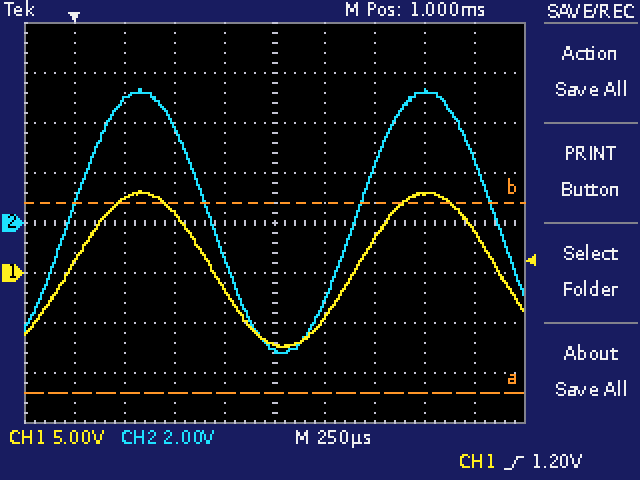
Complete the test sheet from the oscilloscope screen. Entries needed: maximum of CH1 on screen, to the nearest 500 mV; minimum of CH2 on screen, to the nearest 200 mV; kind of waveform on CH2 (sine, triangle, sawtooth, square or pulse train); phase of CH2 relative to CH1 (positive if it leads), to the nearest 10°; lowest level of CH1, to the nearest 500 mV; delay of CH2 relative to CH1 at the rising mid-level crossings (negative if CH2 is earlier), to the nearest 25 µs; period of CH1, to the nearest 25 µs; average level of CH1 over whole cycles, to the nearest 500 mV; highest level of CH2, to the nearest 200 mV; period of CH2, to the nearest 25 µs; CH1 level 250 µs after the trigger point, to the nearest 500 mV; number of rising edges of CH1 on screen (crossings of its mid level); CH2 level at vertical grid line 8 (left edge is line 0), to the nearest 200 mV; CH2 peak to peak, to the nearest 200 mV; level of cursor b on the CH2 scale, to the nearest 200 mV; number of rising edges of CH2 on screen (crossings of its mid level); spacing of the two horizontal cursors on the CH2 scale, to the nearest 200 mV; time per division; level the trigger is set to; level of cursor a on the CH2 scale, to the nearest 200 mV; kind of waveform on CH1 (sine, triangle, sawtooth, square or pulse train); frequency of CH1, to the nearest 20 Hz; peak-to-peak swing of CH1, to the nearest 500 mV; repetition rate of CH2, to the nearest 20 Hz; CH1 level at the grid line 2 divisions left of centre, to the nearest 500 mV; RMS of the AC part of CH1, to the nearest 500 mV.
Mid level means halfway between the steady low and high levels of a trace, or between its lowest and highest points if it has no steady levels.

8.0 V
-5.2 V
sine
0°
-7.5 V
0 µs
1.425 ms
500 mV
5.4 V
1.425 ms
7.5 V
2
5.2 V
10.6 V
800 mV
2
7.6 V
250 µs
1.20 V
-6.8 V
sine
700 Hz
15.5 V
700 Hz
6.0 V
5.5 V
